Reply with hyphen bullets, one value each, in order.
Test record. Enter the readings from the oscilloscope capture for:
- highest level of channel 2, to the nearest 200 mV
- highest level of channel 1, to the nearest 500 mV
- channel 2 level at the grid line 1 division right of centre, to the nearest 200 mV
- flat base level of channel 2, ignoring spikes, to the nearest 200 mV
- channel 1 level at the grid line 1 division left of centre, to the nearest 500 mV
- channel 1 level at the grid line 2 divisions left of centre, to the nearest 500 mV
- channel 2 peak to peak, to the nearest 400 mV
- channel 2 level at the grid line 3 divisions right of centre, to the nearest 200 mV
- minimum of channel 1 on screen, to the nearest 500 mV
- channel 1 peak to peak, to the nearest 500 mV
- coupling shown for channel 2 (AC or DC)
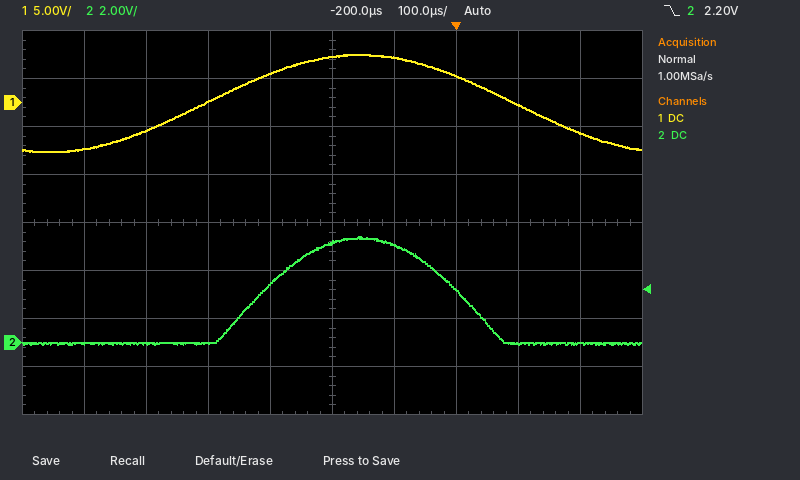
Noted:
- 4.4 V
- 5.0 V
- 4.0 V
- 0.0 V
- 3.0 V
- 0.0 V
- 4.4 V
- 0.0 V
- -5.0 V
- 10.0 V
- DC
